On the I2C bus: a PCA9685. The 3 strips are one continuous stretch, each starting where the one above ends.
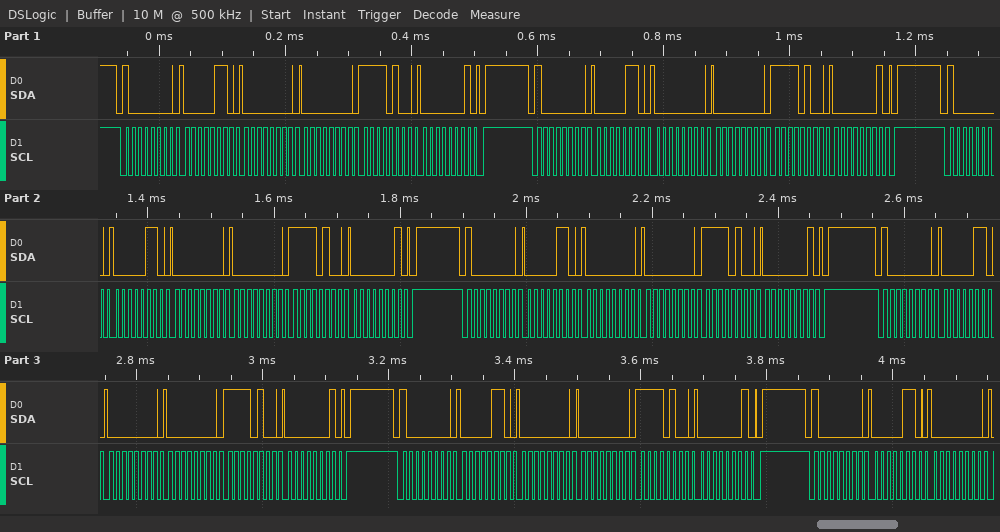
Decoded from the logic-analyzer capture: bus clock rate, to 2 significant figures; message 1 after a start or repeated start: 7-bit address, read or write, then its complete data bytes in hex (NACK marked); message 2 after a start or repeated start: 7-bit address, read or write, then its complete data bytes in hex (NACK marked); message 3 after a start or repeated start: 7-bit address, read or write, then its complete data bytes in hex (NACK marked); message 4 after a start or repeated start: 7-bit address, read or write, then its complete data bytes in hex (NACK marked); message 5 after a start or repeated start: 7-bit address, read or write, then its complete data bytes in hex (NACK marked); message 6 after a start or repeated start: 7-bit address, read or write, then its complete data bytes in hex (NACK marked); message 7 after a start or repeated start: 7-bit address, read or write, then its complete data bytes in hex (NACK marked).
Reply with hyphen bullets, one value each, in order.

- 100 kHz
- 0x40 write: 06 00 00 F4 01
- 0x40 write: 06 00 00 F4 01
- 0x40 write: 06 00 00 F4 01
- 0x40 write: 06 00 00 F4 01
- 0x40 write: 06 00 00 F4 01
- 0x40 write: 06 00 00 F4 01
- 0x40 write: 06 00
